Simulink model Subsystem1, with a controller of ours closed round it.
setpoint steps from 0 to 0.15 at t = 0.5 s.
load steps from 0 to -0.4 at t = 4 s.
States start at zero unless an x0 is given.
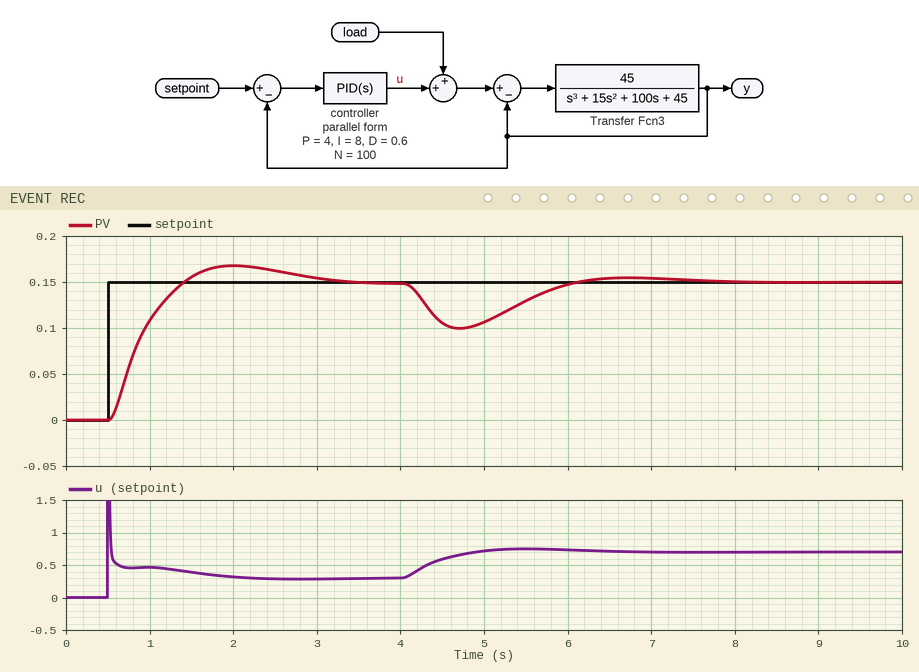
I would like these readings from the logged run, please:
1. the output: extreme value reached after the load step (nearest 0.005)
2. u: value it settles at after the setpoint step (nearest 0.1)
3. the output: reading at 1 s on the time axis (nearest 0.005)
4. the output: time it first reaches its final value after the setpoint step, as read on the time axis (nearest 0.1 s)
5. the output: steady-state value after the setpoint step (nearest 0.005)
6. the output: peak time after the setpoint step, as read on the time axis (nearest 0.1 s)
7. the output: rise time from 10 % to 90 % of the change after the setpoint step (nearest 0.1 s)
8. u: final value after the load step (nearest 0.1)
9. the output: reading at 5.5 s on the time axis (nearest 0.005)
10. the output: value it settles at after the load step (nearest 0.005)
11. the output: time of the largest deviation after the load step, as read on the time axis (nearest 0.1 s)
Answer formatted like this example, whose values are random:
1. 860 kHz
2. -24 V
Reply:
1. 0.100
2. 0.3
3. 0.110
4. 1.4 s
5. 0.150
6. 2.0 s
7. 0.6 s
8. 0.7
9. 0.130
10. 0.150
11. 4.7 s
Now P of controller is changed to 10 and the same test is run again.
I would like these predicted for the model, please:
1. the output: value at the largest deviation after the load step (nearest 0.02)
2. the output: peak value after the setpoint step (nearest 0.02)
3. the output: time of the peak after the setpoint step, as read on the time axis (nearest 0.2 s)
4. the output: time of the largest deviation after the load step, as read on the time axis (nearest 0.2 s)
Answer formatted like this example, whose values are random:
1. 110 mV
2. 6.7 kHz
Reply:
1. 0.12
2. 0.16
3. 1.0 s
4. 4.6 s
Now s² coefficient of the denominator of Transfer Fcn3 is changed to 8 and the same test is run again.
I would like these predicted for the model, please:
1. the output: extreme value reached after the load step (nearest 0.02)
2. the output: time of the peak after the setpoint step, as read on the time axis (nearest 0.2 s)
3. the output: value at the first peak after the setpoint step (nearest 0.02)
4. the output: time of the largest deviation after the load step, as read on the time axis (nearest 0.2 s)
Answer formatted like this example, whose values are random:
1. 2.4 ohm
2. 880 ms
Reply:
1. 0.10
2. 2.2 s
3. 0.16
4. 4.6 s
